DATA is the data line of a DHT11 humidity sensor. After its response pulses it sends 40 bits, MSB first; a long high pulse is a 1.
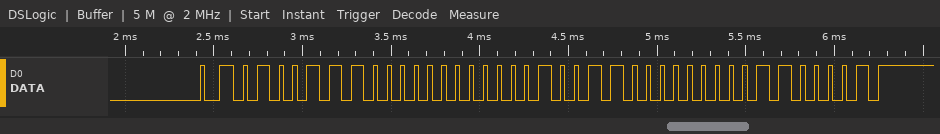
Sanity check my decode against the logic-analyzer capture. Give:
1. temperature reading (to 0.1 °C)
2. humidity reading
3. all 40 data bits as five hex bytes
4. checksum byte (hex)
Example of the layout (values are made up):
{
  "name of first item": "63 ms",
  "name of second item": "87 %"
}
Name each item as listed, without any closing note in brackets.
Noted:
{
  "temperature reading": "19.0 °C",
  "humidity reading": "78 %",
  "all 40 data bits as five hex bytes": "4E 00 13 00 61",
  "checksum byte": "0x61"
}
